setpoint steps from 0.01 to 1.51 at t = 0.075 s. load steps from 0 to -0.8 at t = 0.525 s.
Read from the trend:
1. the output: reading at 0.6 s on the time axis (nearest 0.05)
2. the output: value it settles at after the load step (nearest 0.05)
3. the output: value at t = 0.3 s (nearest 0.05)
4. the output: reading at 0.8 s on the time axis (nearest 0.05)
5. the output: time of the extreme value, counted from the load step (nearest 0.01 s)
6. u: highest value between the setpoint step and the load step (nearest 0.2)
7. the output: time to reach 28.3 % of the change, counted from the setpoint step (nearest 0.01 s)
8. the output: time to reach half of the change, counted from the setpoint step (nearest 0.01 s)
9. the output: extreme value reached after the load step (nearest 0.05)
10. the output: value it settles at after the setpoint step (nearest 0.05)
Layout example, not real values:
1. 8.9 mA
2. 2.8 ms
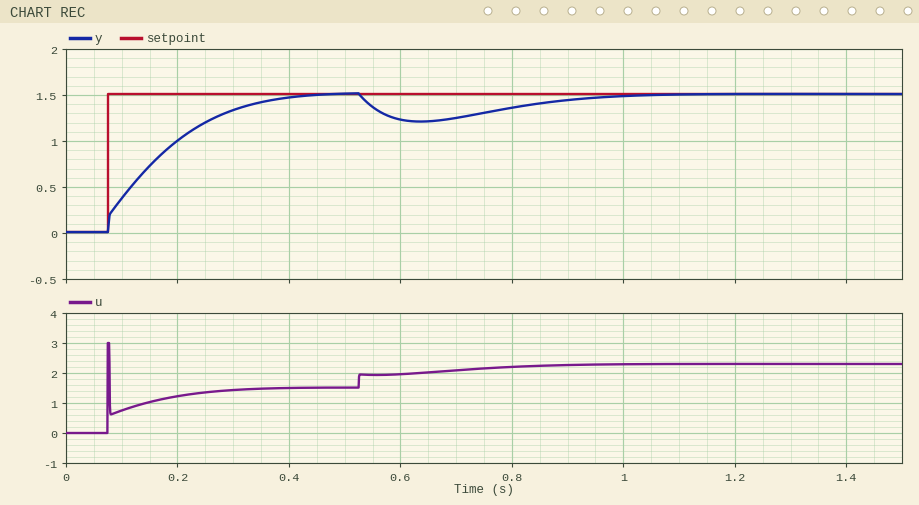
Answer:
1. 1.25
2. 1.50
3. 1.35
4. 1.35
5. 0.11 s
6. 3.0
7. 0.03 s
8. 0.08 s
9. 1.20
10. 1.50
